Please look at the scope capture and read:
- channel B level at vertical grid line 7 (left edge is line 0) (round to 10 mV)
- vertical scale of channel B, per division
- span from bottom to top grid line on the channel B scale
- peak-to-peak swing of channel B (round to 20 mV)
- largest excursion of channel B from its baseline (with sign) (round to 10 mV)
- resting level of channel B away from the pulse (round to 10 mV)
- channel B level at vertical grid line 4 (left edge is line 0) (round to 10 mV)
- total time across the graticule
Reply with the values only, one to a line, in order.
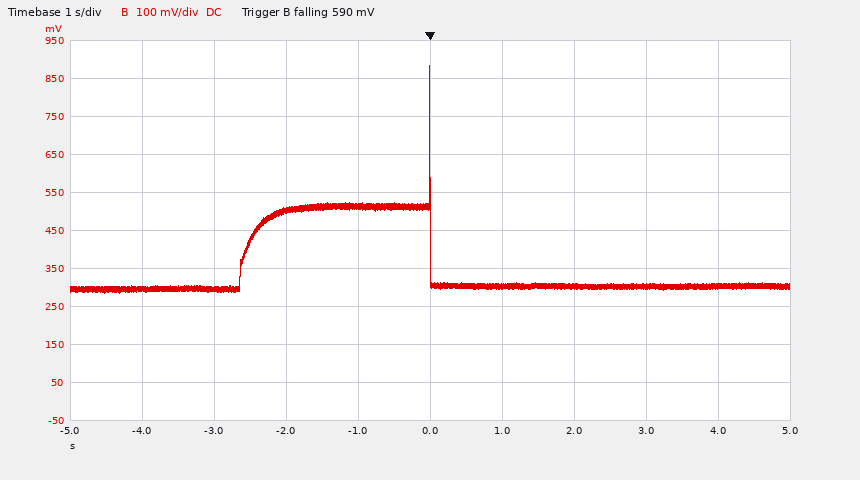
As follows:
300 mV
100 mV
1 V
600 mV
+580 mV
300 mV
510 mV
10 s
